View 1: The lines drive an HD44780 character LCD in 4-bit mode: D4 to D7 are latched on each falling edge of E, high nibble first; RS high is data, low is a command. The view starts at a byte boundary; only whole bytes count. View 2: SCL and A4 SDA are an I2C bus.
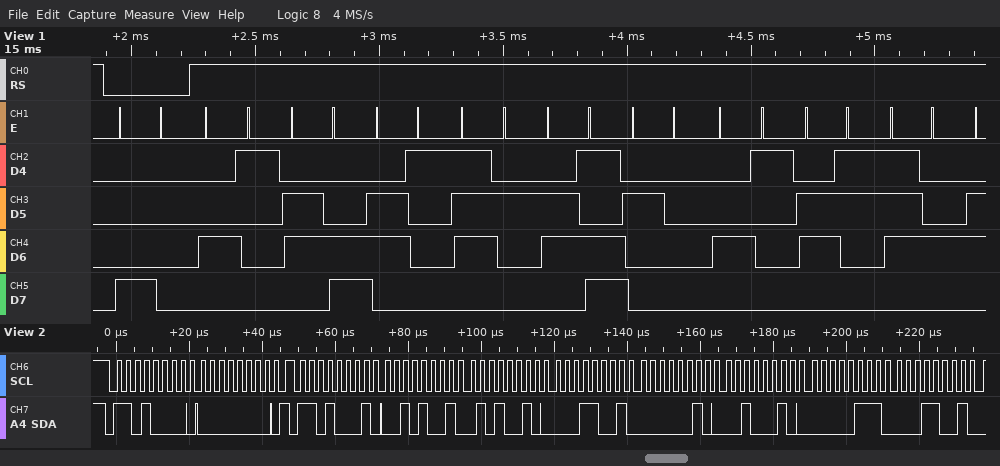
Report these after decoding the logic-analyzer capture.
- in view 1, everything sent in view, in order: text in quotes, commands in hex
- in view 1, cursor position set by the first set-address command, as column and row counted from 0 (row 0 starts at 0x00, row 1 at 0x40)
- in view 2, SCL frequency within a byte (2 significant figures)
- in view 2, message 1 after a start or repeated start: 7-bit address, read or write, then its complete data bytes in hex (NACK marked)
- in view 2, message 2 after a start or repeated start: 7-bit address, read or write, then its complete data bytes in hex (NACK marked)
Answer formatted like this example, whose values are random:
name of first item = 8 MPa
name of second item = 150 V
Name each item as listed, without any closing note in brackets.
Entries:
in view 1, everything sent in view, in order: text in quotes, commands in hex = 0x80 "Alarm Act"
in view 1, cursor position set by the first set-address command, as column and row counted from 0 = column 0, row 0
in view 2, SCL frequency within a byte = 400 kHz
in view 2, message 1 after a start or repeated start: 7-bit address, read or write, then its complete data bytes in hex = 0x68 write: 00
in view 2, message 2 after a start or repeated start: 7-bit address, read or write, then its complete data bytes in hex = 0x68 read: 29 52 19 02 22 07 19
